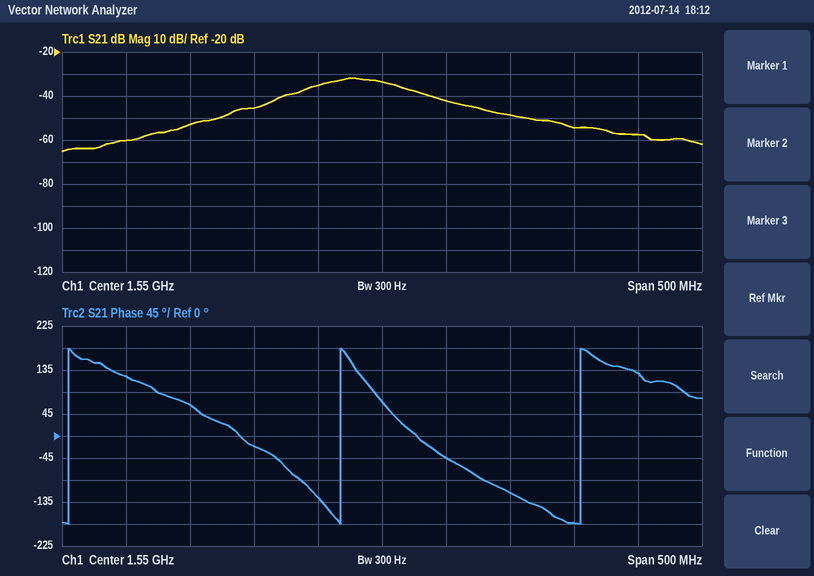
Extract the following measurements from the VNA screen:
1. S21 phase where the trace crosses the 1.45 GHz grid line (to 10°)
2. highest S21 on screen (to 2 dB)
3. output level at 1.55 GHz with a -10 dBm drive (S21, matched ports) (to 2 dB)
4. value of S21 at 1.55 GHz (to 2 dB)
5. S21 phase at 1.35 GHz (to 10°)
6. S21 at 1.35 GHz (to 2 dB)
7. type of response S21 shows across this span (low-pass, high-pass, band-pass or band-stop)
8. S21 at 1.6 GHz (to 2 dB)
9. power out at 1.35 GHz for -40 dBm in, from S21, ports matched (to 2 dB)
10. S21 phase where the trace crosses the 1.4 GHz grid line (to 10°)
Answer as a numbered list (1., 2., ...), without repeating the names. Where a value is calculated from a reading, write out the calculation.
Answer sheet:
1. -20°
2. -32 dB
3. -10 dBm + (-34 dB) = -44 dBm
4. -34 dB
5. 120°
6. -60 dB
7. band-pass
8. -42 dB
9. -40 dBm + (-60 dB) = -100 dBm
10. 60°
